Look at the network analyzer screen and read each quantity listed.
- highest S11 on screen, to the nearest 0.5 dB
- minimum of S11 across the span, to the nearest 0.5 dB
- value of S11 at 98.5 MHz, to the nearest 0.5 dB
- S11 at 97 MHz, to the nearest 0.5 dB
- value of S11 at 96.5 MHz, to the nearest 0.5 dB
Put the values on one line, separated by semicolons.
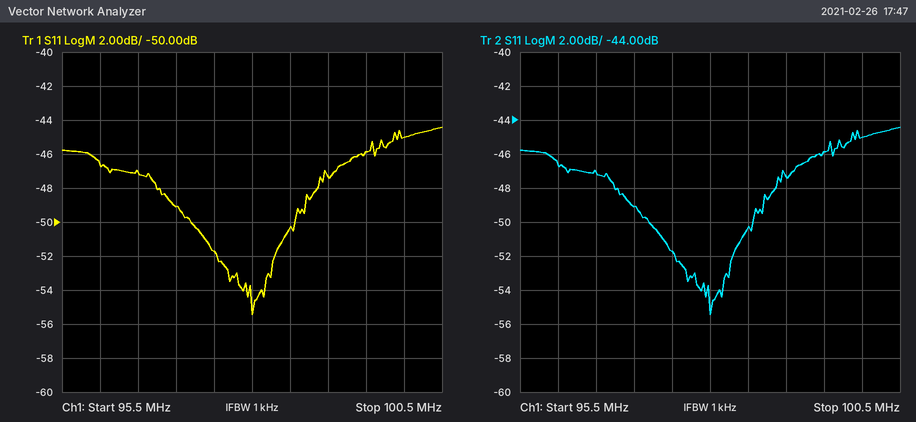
-44.5 dB; -55.5 dB; -50.5 dB; -49.0 dB; -47.0 dB
